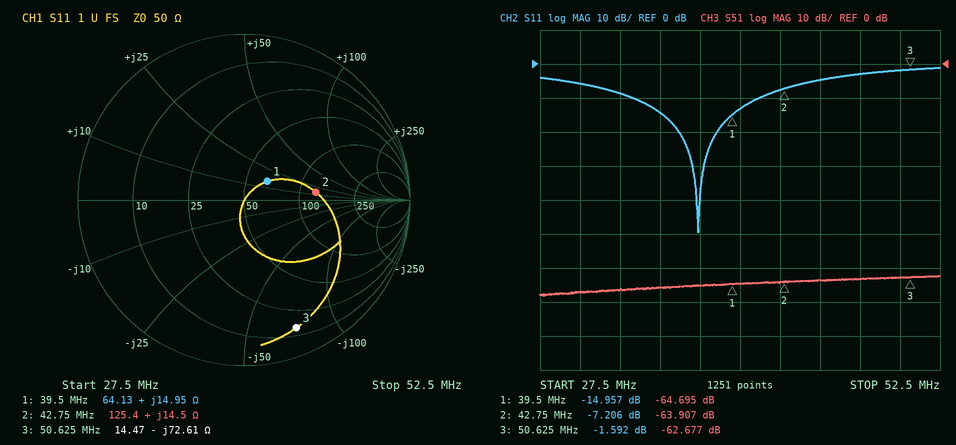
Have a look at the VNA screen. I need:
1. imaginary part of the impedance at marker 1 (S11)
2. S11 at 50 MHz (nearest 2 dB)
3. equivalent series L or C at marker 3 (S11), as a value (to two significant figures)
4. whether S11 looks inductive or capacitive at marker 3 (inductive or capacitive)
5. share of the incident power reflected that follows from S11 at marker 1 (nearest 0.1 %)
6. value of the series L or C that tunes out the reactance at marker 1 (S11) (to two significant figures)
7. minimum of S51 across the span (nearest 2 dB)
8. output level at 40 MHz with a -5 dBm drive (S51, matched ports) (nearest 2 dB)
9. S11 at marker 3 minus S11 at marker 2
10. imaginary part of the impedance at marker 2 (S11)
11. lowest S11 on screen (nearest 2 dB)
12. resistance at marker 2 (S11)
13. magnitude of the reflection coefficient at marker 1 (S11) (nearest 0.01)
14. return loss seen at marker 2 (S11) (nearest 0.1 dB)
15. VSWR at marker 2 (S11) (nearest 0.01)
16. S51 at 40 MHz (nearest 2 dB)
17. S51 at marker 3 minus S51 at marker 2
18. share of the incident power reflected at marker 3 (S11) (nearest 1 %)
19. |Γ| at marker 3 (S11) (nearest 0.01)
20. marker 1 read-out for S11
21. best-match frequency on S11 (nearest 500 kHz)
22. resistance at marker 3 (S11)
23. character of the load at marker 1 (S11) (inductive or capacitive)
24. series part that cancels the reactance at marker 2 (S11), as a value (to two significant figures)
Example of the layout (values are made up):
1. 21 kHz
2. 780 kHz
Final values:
1. +14.95 Ω
2. -2 dB
3. 43 pF
4. capacitive
5. 3.2 %
6. 270 pF
7. -68 dB
8. -70 dBm
9. 5.614 dB
10. +14.5 Ω
11. -50 dB
12. 125.4 Ω
13. 0.18
14. 7.2 dB
15. 2.55
16. -64 dB
17. 1.230 dB
18. 69 %
19. 0.83
20. -14.957 dB
21. 37.5 MHz
22. 14.47 Ω
23. inductive
24. 260 pF
